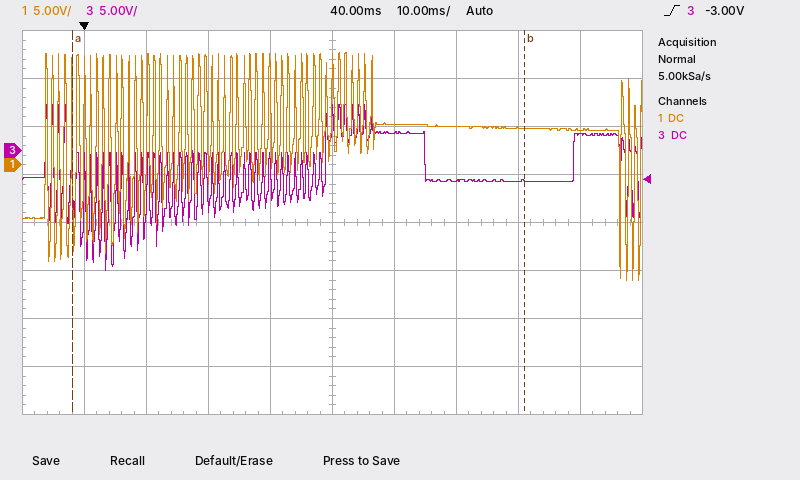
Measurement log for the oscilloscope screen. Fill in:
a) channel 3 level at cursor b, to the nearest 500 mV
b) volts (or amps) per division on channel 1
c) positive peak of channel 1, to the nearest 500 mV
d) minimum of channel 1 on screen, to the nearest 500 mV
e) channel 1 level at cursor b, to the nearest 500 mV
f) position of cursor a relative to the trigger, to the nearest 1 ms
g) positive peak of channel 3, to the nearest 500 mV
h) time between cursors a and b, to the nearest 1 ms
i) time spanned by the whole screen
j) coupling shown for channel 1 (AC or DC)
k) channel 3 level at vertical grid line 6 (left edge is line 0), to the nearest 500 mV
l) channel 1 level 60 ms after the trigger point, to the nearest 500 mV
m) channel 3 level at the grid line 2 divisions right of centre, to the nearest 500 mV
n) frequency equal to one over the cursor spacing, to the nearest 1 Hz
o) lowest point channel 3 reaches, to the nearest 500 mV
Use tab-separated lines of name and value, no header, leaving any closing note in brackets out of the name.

channel 3 level at cursor b, to the nearest 500 mV	-3.0 V
volts (or amps) per division on channel 1	5 V
positive peak of channel 1, to the nearest 500 mV	11.5 V
minimum of channel 1 on screen, to the nearest 500 mV	-12.0 V
channel 1 level at cursor b, to the nearest 500 mV	4.0 V
position of cursor a relative to the trigger, to the nearest 1 ms	-2 ms
positive peak of channel 3, to the nearest 500 mV	5.0 V
time between cursors a and b, to the nearest 1 ms	73 ms
time spanned by the whole screen	100 ms
coupling shown for channel 1	DC
channel 3 level at vertical grid line 6 (left edge is line 0), to the nearest 500 mV	2.0 V
channel 1 level 60 ms after the trigger point, to the nearest 500 mV	4.0 V
channel 3 level at the grid line 2 divisions right of centre, to the nearest 500 mV	-3.0 V
frequency equal to one over the cursor spacing, to the nearest 1 Hz	14 Hz
lowest point channel 3 reaches, to the nearest 500 mV	-12.5 V
